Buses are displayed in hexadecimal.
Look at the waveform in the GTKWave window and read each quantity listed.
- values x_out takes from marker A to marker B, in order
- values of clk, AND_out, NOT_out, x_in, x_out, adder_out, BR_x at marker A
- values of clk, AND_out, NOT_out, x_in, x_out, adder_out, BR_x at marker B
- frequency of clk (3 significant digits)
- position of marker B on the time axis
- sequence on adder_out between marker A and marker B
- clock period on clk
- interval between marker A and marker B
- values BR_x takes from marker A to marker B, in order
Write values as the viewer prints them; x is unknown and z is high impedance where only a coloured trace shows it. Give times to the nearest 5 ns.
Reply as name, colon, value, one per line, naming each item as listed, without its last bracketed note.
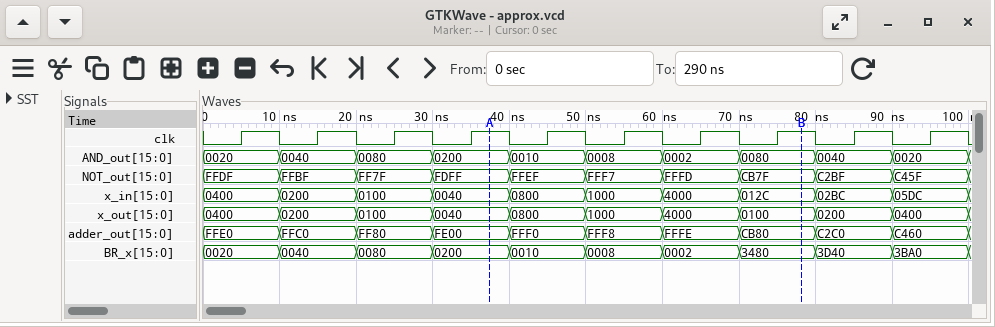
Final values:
values x_out takes from marker A to marker B, in order: 0040, 0800, 1000, 4000, 0100
values of clk, AND_out, NOT_out, x_in, x_out, adder_out, BR_x at marker A: clk=1, AND_out=0200, NOT_out=FDFF, x_in=0040, x_out=0040, adder_out=FE00, BR_x=0200
values of clk, AND_out, NOT_out, x_in, x_out, adder_out, BR_x at marker B: clk=1, AND_out=0080, NOT_out=CB7F, x_in=012C, x_out=0100, adder_out=CB80, BR_x=3480
frequency of clk: 100 MHz
position of marker B on the time axis: 80 ns
sequence on adder_out between marker A and marker B: FE00, FFF0, FFF8, FFFE, CB80
clock period on clk: 10 ns
interval between marker A and marker B: 40 ns
values BR_x takes from marker A to marker B, in order: 0200, 0010, 0008, 0002, 3480
